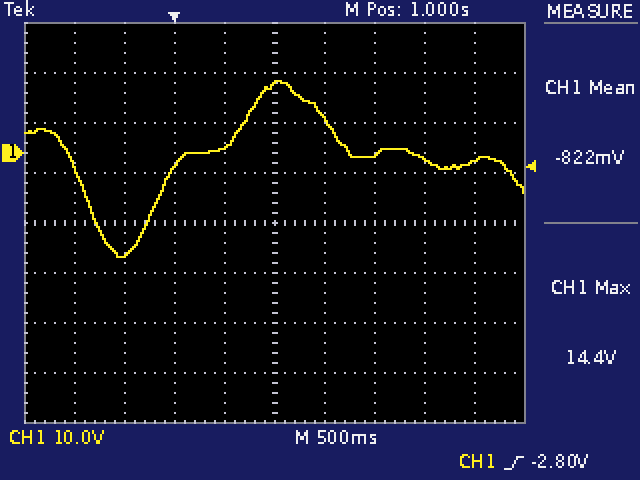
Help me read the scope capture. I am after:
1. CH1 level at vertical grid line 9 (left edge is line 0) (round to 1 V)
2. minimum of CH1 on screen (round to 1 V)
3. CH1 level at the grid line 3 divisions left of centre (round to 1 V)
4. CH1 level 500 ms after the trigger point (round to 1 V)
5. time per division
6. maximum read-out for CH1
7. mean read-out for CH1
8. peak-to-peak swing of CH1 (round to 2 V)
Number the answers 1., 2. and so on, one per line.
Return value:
1. -2 V
2. -21 V
3. -20 V
4. 1 V
5. 500 ms
6. 14.4 V
7. -822 mV
8. 36 V
